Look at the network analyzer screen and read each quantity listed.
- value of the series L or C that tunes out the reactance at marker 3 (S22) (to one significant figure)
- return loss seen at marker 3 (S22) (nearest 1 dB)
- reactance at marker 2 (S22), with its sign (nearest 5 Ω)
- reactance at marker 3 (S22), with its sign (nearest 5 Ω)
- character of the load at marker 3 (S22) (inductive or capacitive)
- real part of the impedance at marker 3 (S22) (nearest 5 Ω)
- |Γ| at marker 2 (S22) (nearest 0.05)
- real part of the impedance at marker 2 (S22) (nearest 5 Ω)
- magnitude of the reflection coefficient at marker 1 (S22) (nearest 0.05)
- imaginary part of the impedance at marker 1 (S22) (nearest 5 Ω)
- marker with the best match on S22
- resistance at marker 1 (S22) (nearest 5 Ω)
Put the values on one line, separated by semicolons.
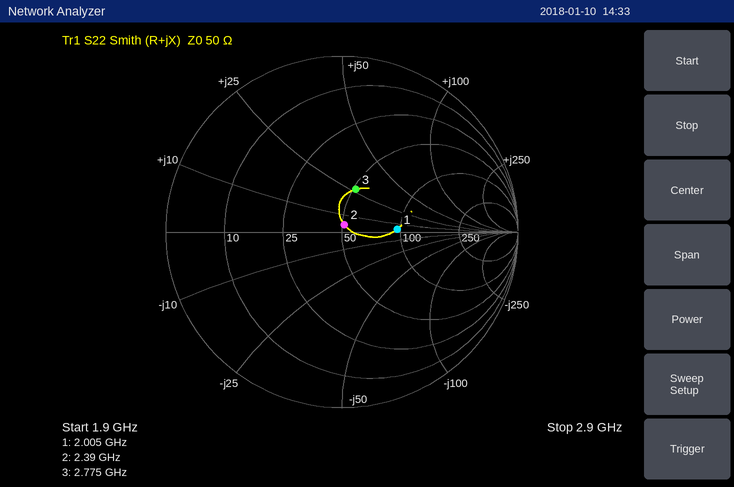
2 pF; 12 dB; +5 Ω; +25 Ω; inductive; 50 Ω; 0.05; 50 Ω; 0.30; +5 Ω; marker 2; 95 Ω
